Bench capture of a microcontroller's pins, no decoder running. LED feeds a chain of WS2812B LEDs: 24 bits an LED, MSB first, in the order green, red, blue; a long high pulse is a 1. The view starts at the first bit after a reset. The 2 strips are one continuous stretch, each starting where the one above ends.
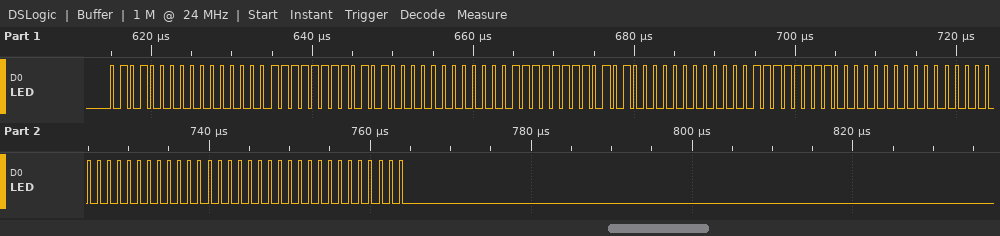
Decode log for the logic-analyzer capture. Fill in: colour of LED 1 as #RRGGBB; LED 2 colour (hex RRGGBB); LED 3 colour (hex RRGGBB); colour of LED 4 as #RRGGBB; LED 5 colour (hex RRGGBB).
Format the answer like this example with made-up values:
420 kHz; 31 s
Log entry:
#0050FF; #0050FF; #0050FF; #000000; #000000
